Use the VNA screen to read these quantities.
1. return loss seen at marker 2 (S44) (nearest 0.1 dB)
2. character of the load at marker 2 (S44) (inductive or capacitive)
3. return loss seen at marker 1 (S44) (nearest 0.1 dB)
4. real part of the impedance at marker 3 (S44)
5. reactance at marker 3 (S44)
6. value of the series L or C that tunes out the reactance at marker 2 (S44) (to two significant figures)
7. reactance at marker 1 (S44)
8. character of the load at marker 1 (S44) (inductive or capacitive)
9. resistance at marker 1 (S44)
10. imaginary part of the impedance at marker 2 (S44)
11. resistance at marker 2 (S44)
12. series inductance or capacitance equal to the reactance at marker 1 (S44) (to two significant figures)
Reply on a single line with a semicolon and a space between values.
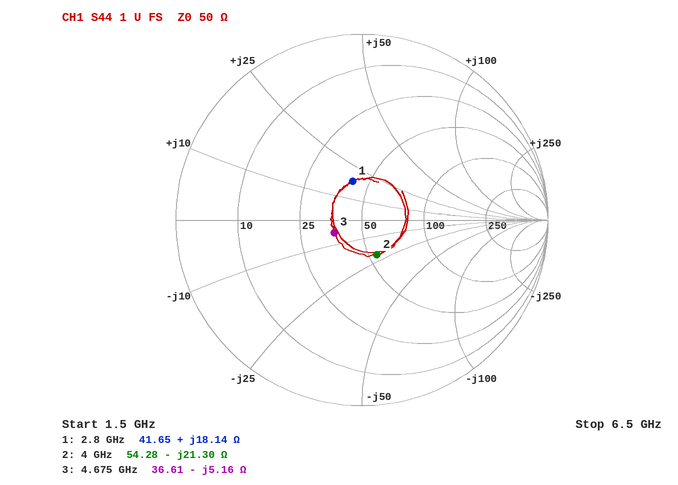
13.8 dB; capacitive; 13.4 dB; 36.61 Ω; -5.16 Ω; 850 pH; +18.14 Ω; inductive; 41.65 Ω; -21.30 Ω; 54.28 Ω; 1.0 nH
